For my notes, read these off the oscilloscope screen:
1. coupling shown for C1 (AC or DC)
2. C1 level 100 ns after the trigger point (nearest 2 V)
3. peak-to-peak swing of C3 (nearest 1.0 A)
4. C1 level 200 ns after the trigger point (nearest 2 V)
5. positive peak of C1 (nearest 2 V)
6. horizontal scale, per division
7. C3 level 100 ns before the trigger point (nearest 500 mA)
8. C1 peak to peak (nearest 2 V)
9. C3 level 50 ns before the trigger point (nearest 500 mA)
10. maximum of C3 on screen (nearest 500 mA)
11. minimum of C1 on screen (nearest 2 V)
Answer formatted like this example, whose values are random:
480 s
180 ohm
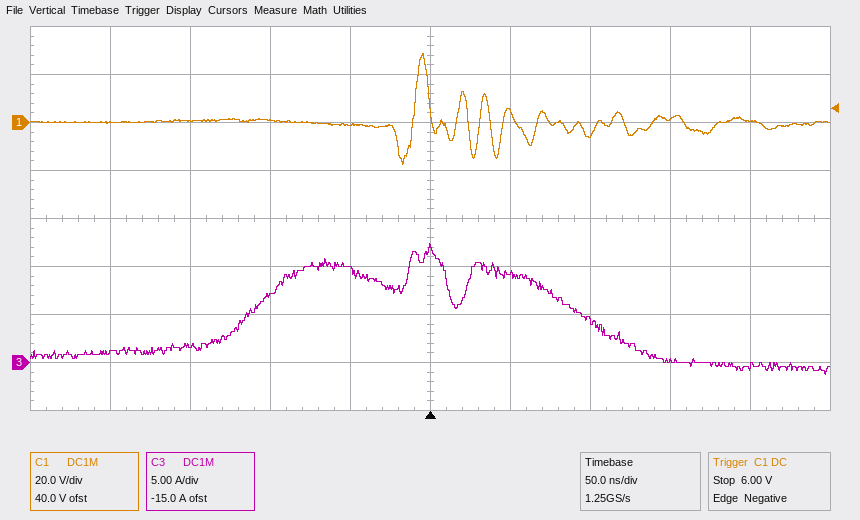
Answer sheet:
DC
-4 V
14.0 A
0 V
28 V
50 ns
7.0 A
46 V
9.5 A
12.5 A
-18 V
